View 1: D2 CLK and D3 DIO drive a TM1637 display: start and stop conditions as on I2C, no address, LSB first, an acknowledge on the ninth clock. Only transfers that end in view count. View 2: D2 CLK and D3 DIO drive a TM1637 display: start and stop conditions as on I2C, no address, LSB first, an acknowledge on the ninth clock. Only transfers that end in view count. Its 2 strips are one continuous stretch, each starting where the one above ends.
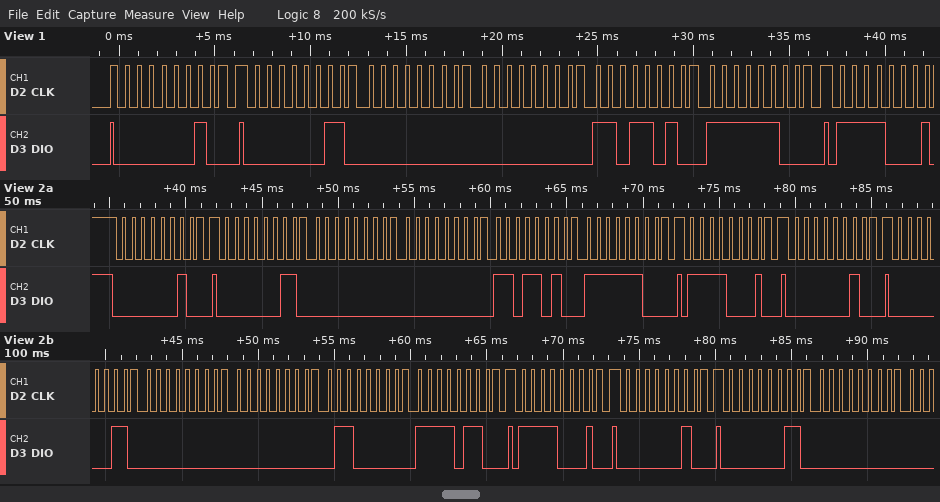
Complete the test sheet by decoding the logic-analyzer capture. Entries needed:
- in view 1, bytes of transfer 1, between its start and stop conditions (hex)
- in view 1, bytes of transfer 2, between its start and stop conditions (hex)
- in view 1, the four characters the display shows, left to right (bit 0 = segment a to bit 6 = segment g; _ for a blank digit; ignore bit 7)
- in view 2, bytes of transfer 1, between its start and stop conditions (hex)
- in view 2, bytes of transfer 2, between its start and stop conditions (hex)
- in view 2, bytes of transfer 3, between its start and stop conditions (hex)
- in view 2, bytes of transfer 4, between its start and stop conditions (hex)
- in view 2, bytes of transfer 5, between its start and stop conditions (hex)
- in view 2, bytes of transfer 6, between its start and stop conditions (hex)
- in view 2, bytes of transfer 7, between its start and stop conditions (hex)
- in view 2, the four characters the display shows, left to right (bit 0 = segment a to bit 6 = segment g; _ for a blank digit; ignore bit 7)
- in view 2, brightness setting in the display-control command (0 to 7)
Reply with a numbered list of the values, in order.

1. 40
2. C0 00 00 5B 3F
3. __20
4. 40
5. C0 00 00 5B 3F
6. 8F
7. 40
8. C0 00 00 06 6F
9. 8F
10. 40
11. __19
12. 7
